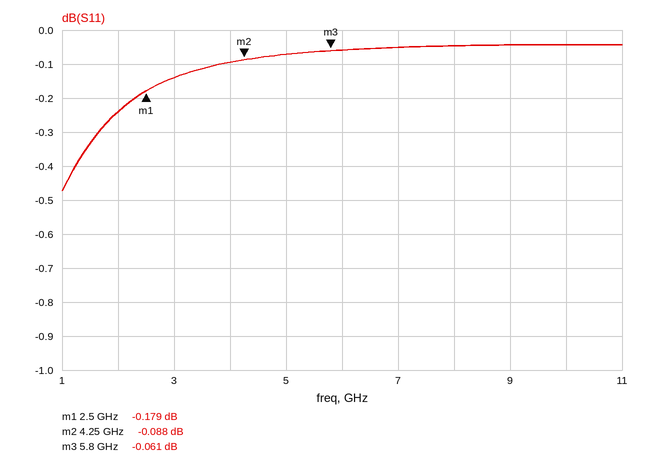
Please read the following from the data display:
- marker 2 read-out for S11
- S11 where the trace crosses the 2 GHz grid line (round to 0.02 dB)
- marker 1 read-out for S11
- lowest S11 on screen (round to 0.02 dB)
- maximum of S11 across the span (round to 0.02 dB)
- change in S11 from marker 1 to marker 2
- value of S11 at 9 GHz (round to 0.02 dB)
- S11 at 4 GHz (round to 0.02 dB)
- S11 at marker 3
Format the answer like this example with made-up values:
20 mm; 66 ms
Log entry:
-0.088 dB; -0.24 dB; -0.179 dB; -0.48 dB; -0.04 dB; 0.091 dB; -0.04 dB; -0.10 dB; -0.061 dB
